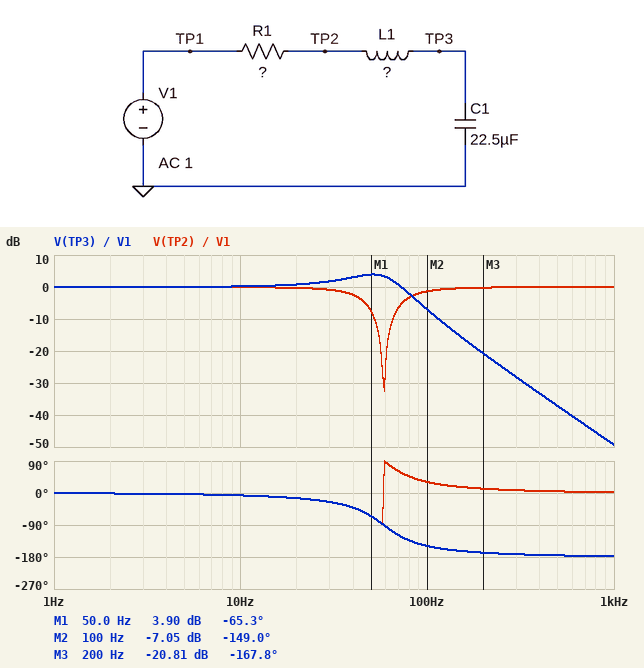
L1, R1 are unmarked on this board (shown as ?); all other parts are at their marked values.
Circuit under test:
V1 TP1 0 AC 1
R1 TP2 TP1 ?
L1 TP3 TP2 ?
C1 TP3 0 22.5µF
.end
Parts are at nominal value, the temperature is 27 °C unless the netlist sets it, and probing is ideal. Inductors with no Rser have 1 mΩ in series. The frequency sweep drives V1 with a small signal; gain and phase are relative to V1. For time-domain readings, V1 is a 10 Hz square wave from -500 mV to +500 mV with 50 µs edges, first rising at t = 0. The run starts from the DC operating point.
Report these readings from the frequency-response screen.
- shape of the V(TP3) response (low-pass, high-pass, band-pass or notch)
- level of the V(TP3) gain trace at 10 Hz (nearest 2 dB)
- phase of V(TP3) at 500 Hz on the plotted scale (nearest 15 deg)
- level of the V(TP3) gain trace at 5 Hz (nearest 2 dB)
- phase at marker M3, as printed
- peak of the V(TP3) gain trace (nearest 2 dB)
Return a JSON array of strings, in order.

["low-pass", "0 dB", "-180 deg", "0 dB", "-167.8 deg", "4 dB"]
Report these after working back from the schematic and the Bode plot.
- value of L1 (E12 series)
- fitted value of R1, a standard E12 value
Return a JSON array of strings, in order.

["330 mH", "82 Ω"]
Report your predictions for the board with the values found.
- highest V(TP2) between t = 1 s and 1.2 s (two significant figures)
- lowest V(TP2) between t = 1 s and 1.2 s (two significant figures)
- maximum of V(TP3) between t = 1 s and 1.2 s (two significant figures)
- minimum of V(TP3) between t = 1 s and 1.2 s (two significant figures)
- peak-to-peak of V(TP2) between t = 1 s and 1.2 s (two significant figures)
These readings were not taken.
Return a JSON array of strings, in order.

["640 mV", "-640 mV", "820 mV", "-820 mV", "1.3 V"]
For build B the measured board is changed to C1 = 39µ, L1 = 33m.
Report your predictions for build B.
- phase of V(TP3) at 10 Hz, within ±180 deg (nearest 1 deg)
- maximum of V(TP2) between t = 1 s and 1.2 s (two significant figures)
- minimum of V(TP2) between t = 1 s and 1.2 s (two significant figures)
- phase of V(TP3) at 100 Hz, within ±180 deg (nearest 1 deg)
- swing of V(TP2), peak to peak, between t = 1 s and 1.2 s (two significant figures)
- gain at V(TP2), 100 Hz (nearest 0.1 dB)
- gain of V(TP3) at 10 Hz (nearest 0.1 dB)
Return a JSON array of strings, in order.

["-11 deg", "500 mV", "-500 mV", "-76 deg", "1.0 V", "-12.5 dB", "-0.1 dB"]
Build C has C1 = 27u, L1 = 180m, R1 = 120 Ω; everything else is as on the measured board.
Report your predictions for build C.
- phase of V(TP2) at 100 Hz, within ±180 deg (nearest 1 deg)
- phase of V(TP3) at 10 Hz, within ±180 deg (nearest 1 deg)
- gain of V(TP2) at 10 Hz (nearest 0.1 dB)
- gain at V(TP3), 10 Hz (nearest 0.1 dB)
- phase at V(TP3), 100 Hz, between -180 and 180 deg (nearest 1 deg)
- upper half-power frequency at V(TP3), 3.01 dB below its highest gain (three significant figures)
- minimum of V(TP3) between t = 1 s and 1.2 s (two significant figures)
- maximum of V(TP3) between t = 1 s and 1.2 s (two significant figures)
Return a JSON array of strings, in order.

["66 deg", "-12 deg", "-0.2 dB", "0 dB", "-114 deg", "69.4 Hz", "-530 mV", "530 mV"]
